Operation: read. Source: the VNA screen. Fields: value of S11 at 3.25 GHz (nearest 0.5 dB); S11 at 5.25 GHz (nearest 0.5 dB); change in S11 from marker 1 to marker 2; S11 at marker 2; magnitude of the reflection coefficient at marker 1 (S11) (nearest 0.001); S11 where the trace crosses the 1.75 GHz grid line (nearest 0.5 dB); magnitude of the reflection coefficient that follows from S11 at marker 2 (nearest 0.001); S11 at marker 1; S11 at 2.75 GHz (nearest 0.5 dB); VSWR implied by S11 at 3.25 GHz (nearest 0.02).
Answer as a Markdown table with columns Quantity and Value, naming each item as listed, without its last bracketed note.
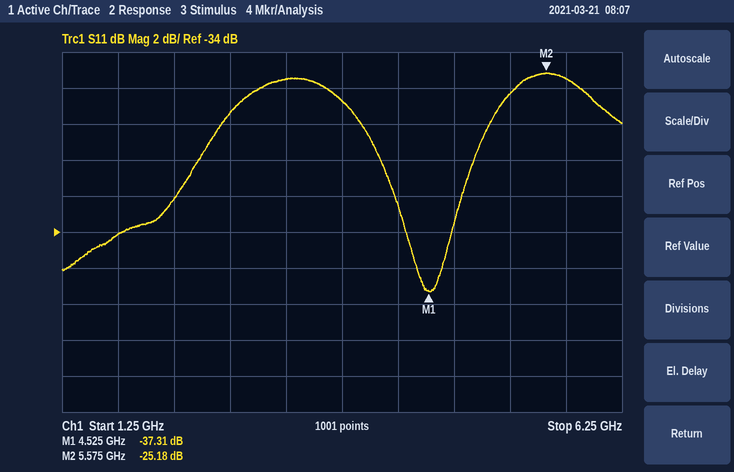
| Quantity | Value |
|---|---|
| value of S11 at 3.25 GHz | -25.5 dB |
| S11 at 5.25 GHz | -26.5 dB |
| change in S11 from marker 1 to marker 2 | 12.13 dB |
| S11 at marker 2 | -25.18 dB |
| magnitude of the reflection coefficient at marker 1 (S11) | 0.014 |
| S11 where the trace crosses the 1.75 GHz grid line | -34.0 dB |
| magnitude of the reflection coefficient that follows from S11 at marker 2 | 0.055 |
| S11 at marker 1 | -37.31 dB |
| S11 at 2.75 GHz | -27.5 dB |
| VSWR implied by S11 at 3.25 GHz | 1.12 |
